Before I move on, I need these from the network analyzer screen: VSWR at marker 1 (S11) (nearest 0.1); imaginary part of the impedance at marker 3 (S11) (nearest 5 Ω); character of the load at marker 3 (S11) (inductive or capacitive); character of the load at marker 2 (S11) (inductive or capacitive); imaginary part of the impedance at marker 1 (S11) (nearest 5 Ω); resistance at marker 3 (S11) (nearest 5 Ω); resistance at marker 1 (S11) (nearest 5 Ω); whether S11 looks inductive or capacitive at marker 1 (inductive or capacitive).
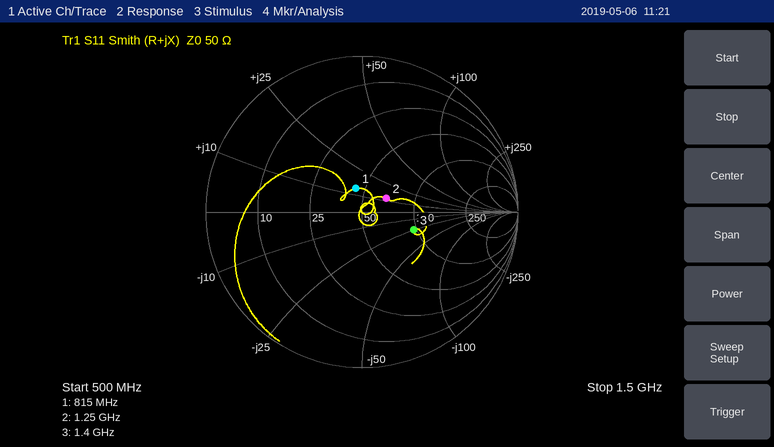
1.4
-25 Ω
capacitive
inductive
+15 Ω
95 Ω
45 Ω
inductive
